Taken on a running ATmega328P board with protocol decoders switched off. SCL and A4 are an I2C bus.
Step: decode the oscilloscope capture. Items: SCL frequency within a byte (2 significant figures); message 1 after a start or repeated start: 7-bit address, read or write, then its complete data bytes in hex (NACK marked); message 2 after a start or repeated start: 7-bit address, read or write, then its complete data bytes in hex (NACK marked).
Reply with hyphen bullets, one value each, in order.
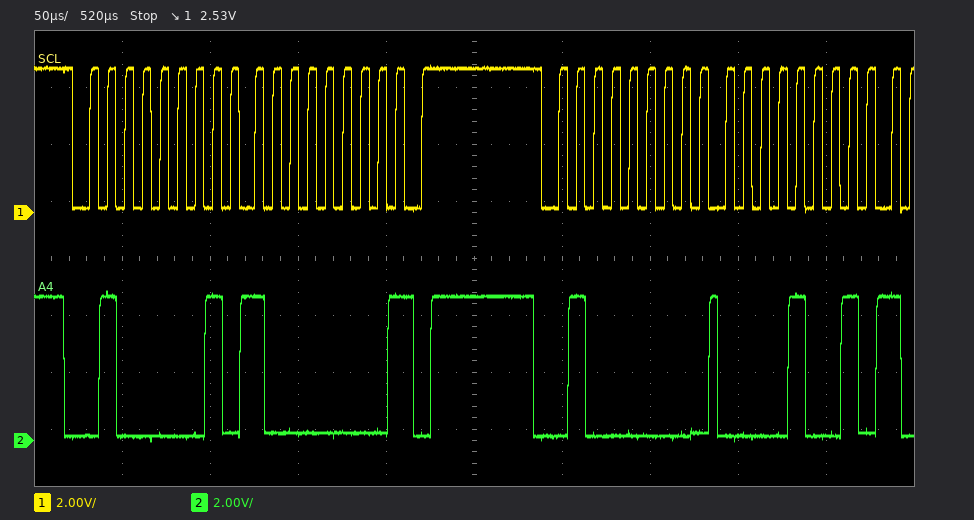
- 100 kHz
- 0x20 read: 80 NACK
- 0x20 write: 09
